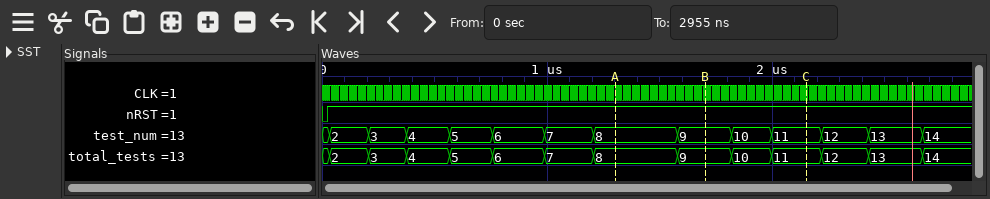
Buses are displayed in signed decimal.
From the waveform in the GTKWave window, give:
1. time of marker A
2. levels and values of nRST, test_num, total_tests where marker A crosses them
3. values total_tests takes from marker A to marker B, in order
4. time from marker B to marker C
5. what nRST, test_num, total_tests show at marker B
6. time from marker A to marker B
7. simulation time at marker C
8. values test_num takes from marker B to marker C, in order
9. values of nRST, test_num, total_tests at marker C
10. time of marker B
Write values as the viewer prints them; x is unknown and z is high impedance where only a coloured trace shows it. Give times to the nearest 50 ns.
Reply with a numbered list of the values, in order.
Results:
1. 1300 ns
2. nRST=1, test_num=8, total_tests=8
3. 8, 9
4. 450 ns
5. nRST=1, test_num=9, total_tests=9
6. 400 ns
7. 2150 ns
8. 9, 10, 11
9. nRST=1, test_num=11, total_tests=11
10. 1700 ns
